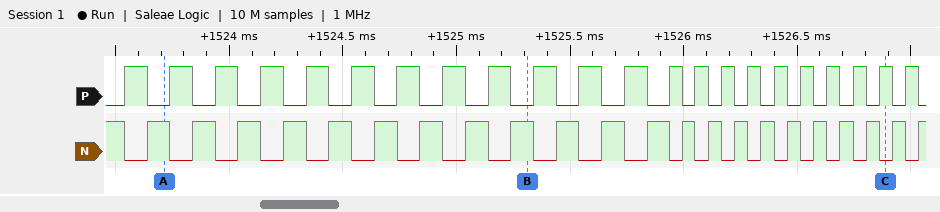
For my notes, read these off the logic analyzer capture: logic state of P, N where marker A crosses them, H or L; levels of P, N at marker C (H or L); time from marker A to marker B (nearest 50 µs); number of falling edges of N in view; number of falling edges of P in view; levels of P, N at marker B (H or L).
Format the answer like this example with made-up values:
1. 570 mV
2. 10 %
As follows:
1. P=L, N=H
2. P=H, N=L
3. 1600 µs
4. 22
5. 22
6. P=L, N=H
